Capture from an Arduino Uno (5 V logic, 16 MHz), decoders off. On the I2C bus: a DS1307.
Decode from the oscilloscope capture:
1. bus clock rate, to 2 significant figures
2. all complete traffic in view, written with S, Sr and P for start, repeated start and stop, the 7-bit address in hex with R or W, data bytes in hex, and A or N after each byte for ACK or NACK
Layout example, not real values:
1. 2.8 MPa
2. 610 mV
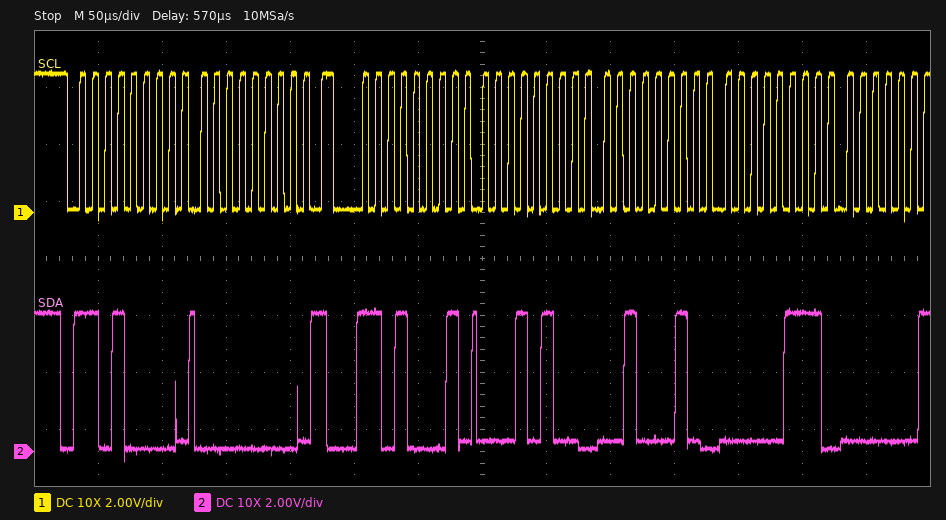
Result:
1. 100 kHz
2. S 68W A 00 A Sr 68R A 14 A 22 A 07 A
